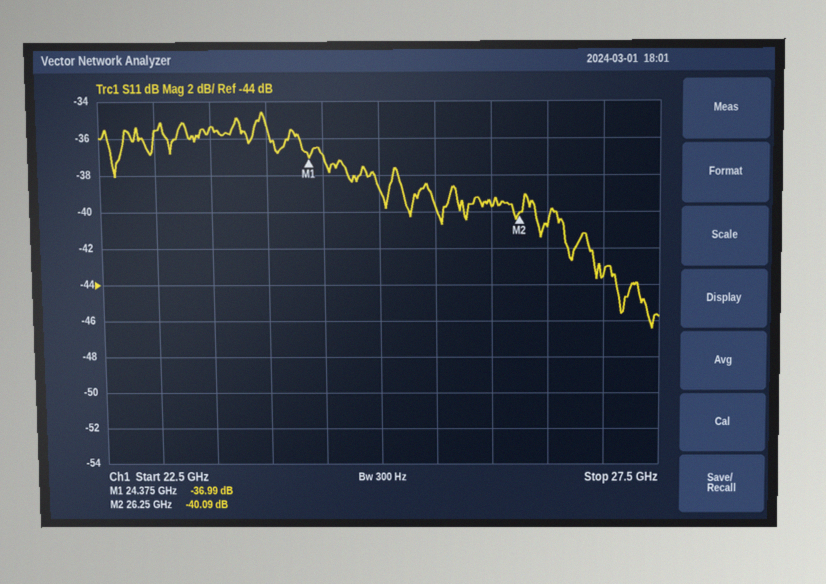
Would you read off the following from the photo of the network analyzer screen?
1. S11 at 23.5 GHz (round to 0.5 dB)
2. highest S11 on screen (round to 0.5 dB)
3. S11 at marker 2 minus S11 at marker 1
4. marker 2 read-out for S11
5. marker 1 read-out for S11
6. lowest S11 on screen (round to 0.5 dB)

-35.5 dB
-34.5 dB
-3.10 dB
-40.09 dB
-36.99 dB
-46.5 dB
